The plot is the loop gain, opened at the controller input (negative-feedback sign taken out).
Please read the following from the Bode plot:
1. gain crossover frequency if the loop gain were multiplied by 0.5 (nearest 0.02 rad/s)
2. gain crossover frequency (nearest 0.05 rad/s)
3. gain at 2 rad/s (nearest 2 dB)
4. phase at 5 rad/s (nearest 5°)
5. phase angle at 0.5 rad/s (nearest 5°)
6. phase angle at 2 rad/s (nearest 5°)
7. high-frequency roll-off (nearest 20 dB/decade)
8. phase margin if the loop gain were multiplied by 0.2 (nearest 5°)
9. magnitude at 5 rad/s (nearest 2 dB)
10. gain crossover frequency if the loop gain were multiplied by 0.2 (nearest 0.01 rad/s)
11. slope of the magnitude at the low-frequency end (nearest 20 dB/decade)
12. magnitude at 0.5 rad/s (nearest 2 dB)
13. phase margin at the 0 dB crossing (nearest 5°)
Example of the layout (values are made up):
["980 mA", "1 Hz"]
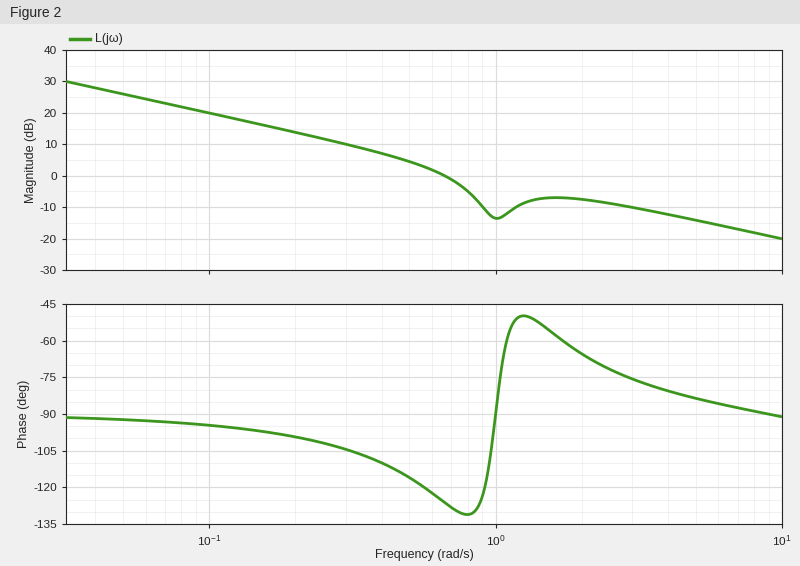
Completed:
["0.44 rad/s", "0.65 rad/s", "-8 dB", "-85°", "-115°", "-65°", "-20 dB/decade", "80°", "-14 dB", "0.20 rad/s", "-20 dB/decade", "4 dB", "55°"]
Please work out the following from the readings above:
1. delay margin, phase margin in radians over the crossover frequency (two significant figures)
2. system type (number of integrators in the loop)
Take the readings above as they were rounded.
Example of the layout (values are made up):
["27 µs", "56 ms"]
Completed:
["1.5 s", "1"]
